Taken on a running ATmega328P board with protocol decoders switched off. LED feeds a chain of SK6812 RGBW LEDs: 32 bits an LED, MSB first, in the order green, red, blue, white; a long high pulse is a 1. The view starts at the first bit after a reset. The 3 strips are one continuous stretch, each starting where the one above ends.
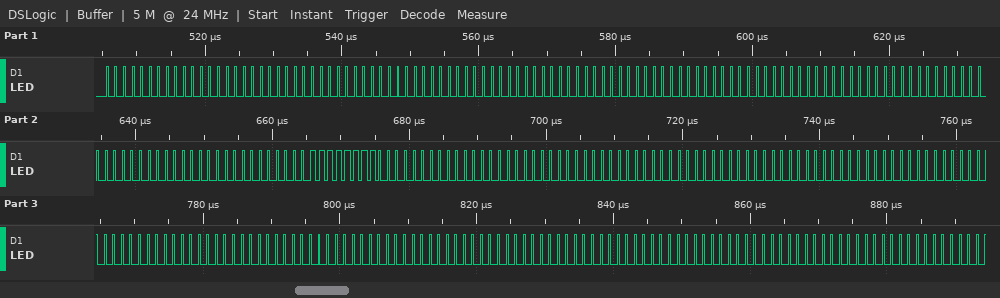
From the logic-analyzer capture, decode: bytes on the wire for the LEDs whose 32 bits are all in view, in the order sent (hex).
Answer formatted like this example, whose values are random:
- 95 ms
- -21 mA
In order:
- 00 00 00 00 00 00 00 00 00 00 00 00 00 00 00 00 FF 00 00 00 00 00 00 00 00 00 00 00 00 00 00 00 00 00 00 00
